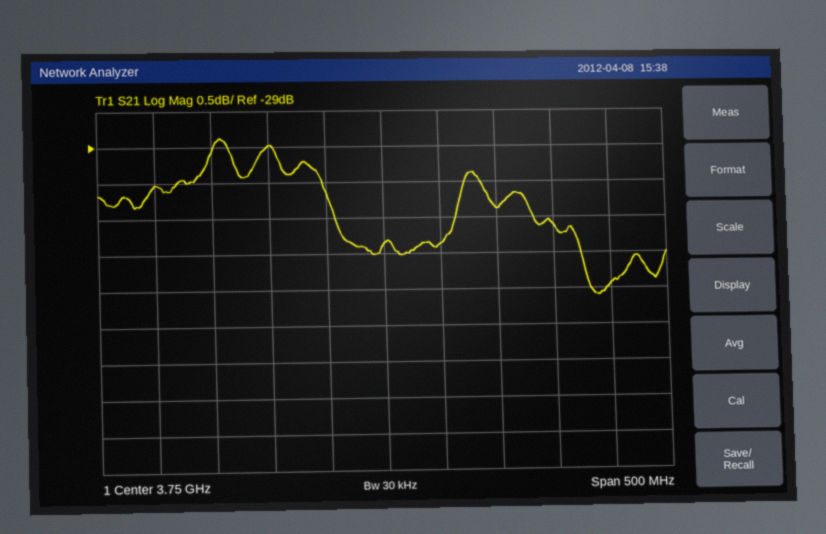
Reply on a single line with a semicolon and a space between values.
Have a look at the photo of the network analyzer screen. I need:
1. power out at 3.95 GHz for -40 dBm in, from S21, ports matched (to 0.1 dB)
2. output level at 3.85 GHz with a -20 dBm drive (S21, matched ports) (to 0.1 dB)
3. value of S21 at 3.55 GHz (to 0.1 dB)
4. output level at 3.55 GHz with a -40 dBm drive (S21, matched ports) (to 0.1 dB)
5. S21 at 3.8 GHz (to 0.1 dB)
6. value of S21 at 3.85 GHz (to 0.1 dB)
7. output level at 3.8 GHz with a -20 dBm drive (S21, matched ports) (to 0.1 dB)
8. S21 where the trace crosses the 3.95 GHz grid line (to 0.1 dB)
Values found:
-70.9 dBm; -49.9 dBm; -29.5 dB; -69.5 dBm; -30.4 dB; -29.9 dB; -50.4 dBm; -30.9 dB
